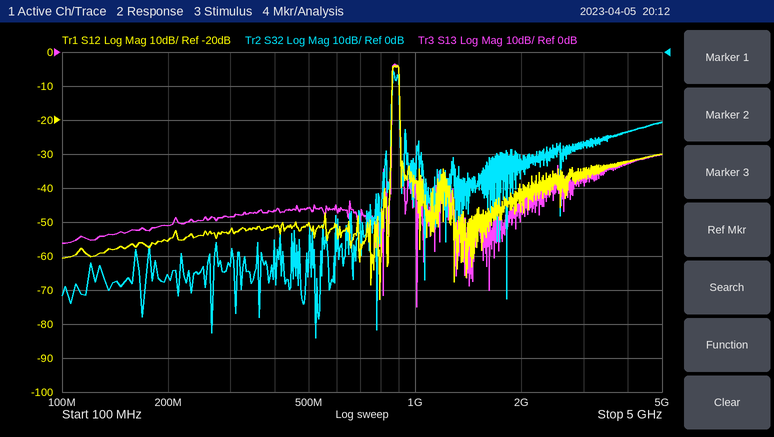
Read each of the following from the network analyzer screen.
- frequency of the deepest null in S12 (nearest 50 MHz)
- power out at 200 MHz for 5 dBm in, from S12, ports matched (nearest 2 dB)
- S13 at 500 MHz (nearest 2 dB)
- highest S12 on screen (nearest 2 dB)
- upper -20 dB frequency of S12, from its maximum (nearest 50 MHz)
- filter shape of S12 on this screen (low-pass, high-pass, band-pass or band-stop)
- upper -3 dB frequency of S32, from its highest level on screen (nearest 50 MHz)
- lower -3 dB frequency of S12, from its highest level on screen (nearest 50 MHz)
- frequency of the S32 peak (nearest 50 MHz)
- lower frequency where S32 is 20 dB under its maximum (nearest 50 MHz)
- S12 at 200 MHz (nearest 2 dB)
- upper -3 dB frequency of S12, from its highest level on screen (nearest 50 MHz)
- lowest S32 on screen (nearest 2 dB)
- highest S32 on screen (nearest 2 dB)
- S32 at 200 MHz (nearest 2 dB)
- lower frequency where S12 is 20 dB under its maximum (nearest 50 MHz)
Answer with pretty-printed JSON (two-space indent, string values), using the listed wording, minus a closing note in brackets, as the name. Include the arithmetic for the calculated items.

{
  "frequency of the deepest null in S12": "800 MHz",
  "power out at 200 MHz for 5 dBm in, from S12, ports matched": "5 dBm + (-56 dB) = -50 dBm",
  "S13 at 500 MHz": "-46 dB",
  "highest S12 on screen": "-4 dB",
  "upper -20 dB frequency of S12, from its maximum": "900 MHz",
  "filter shape of S12 on this screen": "band-pass",
  "upper -3 dB frequency of S32, from its highest level on screen": "900 MHz",
  "lower -3 dB frequency of S12, from its highest level on screen": "850 MHz",
  "frequency of the S32 peak": "850 MHz",
  "lower frequency where S32 is 20 dB under its maximum": "850 MHz",
  "S12 at 200 MHz": "-56 dB",
  "upper -3 dB frequency of S12, from its highest level on screen": "900 MHz",
  "lowest S32 on screen": "-84 dB",
  "highest S32 on screen": "-6 dB",
  "S32 at 200 MHz": "-66 dB",
  "lower frequency where S12 is 20 dB under its maximum": "850 MHz"
}
